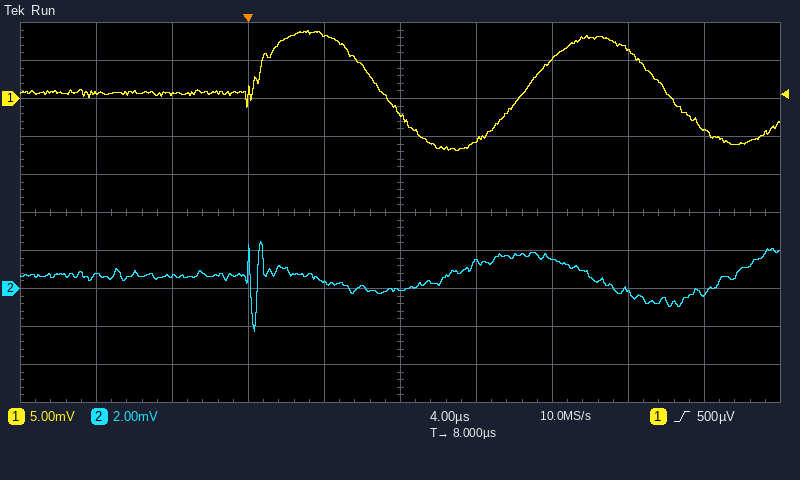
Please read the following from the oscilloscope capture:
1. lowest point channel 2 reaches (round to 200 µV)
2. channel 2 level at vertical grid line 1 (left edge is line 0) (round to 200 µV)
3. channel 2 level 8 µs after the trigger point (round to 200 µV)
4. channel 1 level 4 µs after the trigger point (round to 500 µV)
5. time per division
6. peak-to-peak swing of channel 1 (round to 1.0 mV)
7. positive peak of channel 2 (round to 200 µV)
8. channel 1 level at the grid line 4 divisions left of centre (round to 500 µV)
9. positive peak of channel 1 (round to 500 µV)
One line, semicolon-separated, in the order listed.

-2.2 mV; 600 µV; 0.0 mV; 8.5 mV; 4 µs; 16.0 mV; 2.4 mV; 500 µV; 9.0 mV
